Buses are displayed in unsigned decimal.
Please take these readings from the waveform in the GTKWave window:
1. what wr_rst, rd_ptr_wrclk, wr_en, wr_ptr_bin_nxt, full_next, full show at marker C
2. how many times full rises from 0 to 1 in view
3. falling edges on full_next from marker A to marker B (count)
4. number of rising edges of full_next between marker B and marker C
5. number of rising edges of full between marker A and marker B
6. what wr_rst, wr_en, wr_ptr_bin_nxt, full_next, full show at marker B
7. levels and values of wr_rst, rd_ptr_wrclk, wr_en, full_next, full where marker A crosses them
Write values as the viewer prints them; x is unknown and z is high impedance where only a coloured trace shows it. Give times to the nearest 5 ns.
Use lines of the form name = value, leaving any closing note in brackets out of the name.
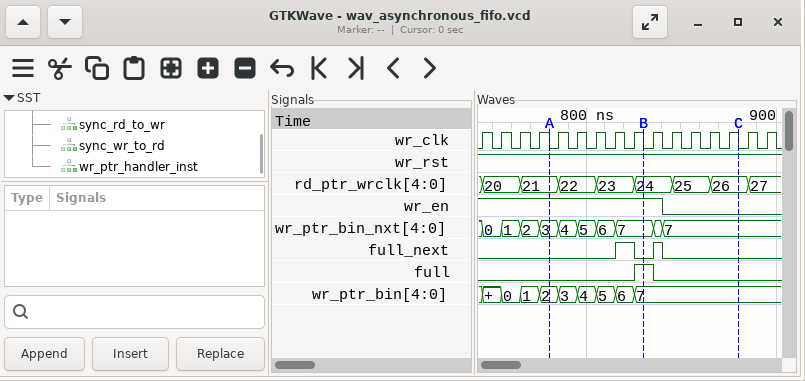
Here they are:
what wr_rst, rd_ptr_wrclk, wr_en, wr_ptr_bin_nxt, full_next, full show at marker C = wr_rst=1, rd_ptr_wrclk=26, wr_en=0, wr_ptr_bin_nxt=7, full_next=0, full=0
how many times full rises from 0 to 1 in view = 1
falling edges on full_next from marker A to marker B = 1
number of rising edges of full_next between marker B and marker C = 1
number of rising edges of full between marker A and marker B = 1
what wr_rst, wr_en, wr_ptr_bin_nxt, full_next, full show at marker B = wr_rst=1, wr_en=1, wr_ptr_bin_nxt=7, full_next=0, full=1
levels and values of wr_rst, rd_ptr_wrclk, wr_en, full_next, full where marker A crosses them = wr_rst=1, rd_ptr_wrclk=21, wr_en=1, full_next=0, full=0
